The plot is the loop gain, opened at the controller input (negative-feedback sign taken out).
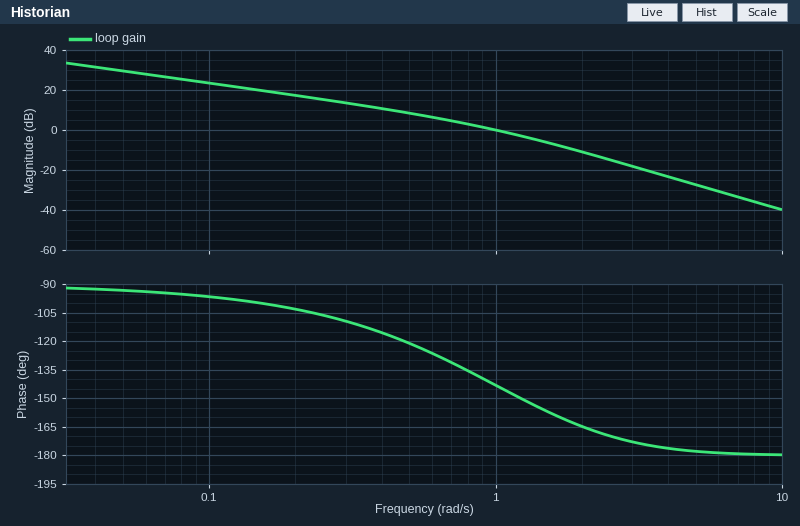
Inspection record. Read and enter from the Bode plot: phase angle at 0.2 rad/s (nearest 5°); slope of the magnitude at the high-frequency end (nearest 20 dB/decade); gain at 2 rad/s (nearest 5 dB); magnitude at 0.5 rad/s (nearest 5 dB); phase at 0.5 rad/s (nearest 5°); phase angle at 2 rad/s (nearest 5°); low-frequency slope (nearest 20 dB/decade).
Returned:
-105°
-40 dB/decade
-10 dB
10 dB
-120°
-165°
-20 dB/decade
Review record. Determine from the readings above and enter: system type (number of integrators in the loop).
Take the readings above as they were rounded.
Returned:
1
